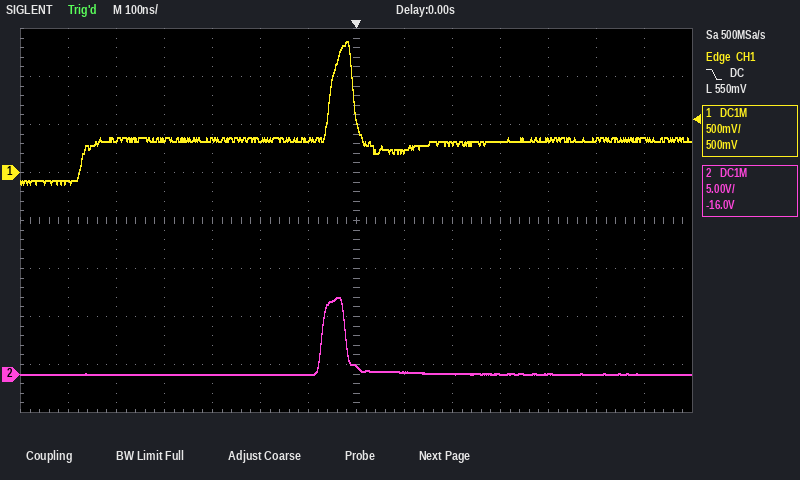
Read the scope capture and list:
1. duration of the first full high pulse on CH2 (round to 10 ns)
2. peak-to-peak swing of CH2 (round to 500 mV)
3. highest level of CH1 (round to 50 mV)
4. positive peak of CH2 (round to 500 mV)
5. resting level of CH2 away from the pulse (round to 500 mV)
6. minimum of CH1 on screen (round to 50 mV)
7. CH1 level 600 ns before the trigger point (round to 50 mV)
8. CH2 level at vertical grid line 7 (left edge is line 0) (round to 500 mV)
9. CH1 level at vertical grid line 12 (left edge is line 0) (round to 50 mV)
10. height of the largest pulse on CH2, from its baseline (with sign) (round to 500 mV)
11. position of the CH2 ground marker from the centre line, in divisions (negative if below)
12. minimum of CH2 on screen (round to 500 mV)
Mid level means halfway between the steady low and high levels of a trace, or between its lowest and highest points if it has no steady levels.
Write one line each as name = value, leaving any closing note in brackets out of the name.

duration of the first full high pulse on CH2 = 50 ns
peak-to-peak swing of CH2 = 8.0 V
highest level of CH1 = 1.35 V
positive peak of CH2 = 8.0 V
resting level of CH2 away from the pulse = 0.0 V
minimum of CH1 on screen = -100 mV
CH1 level 600 ns before the trigger point = -100 mV
CH2 level at vertical grid line 7 (left edge is line 0) = 1.0 V
CH1 level at vertical grid line 12 (left edge is line 0) = 350 mV
height of the largest pulse on CH2, from its baseline (with sign) = +8.0 V
position of the CH2 ground marker from the centre line, in divisions = -3.2 div
minimum of CH2 on screen = 0.0 V
